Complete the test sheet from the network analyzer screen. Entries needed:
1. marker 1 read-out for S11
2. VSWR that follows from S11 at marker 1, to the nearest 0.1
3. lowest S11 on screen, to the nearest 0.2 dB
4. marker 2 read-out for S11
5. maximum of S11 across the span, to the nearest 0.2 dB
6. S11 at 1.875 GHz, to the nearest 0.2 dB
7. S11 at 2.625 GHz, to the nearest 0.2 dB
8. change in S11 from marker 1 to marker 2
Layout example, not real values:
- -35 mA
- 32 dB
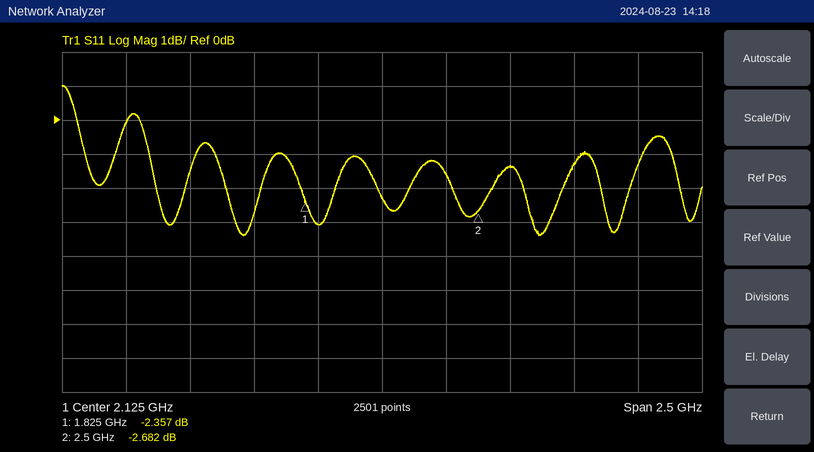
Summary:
- -2.357 dB
- 7.4
- -3.4 dB
- -2.682 dB
- 1.0 dB
- -3.0 dB
- -1.4 dB
- -0.325 dB
